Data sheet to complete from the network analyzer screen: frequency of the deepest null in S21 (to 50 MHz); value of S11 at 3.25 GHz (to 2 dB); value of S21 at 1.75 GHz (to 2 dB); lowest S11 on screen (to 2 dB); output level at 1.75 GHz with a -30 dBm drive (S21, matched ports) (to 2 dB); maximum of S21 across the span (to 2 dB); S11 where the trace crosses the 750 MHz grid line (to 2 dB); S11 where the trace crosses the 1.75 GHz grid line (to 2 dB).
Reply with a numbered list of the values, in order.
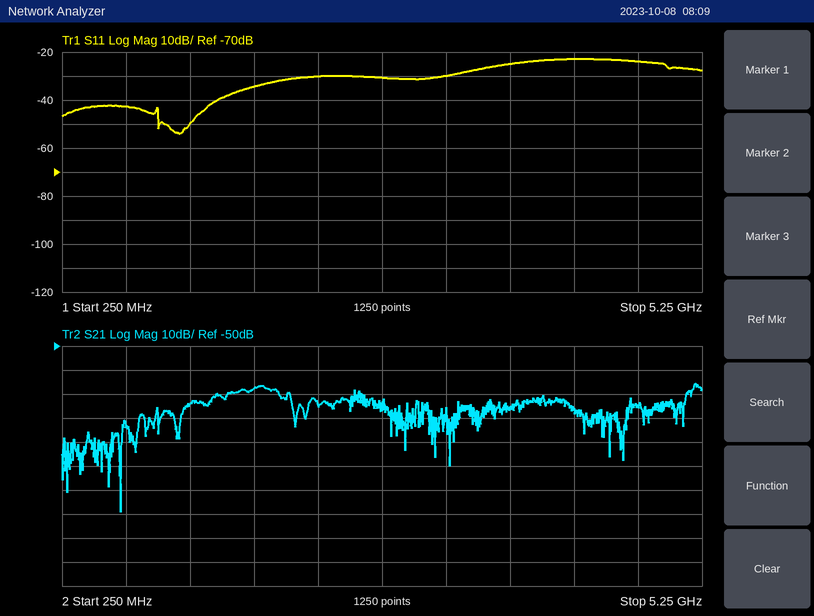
1. 700 MHz
2. -30 dB
3. -68 dB
4. -54 dB
5. -98 dBm
6. -66 dB
7. -42 dB
8. -34 dB
